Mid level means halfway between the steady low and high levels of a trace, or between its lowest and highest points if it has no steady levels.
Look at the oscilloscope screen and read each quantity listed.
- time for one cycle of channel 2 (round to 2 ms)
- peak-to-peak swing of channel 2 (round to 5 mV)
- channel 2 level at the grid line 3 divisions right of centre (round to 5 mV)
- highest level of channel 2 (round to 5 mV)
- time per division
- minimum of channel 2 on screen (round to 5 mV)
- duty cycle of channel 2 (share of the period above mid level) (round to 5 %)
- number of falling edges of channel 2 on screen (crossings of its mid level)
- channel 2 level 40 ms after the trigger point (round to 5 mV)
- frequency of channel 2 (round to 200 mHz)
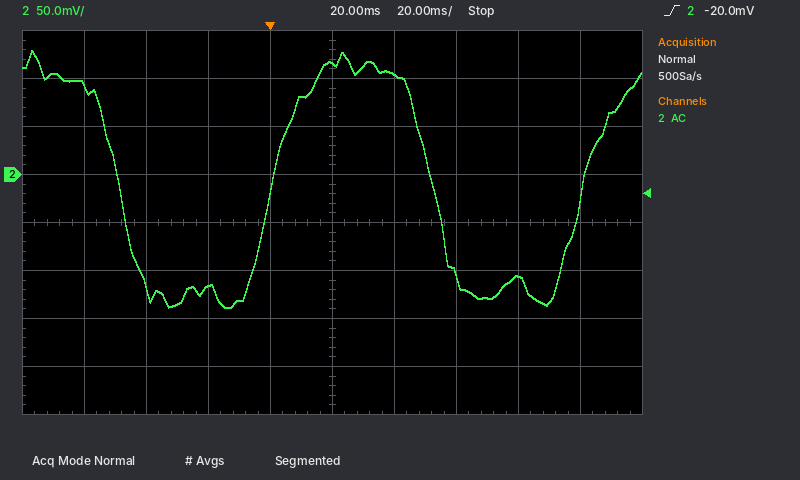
100 ms
270 mV
-105 mV
130 mV
20 ms
-140 mV
50 %
2
105 mV
10.0 Hz
